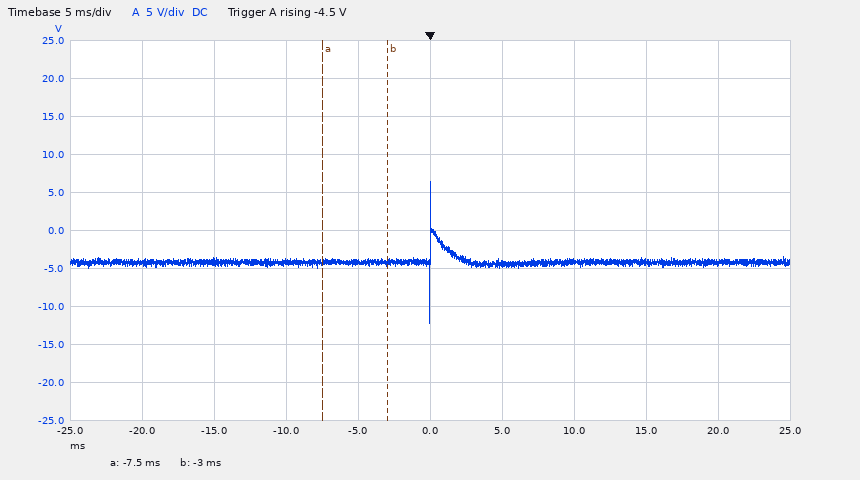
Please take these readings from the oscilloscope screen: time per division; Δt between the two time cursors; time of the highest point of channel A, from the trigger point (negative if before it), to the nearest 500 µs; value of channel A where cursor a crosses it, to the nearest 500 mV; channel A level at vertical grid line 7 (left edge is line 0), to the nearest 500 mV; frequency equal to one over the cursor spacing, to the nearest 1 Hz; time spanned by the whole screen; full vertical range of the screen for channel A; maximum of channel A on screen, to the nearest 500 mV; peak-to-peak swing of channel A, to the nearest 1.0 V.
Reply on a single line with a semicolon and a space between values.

5 ms; 4.5 ms; 0.0 ms; -4.0 V; -4.0 V; 222 Hz; 50 ms; 50 V; 6.5 V; 19.0 V
